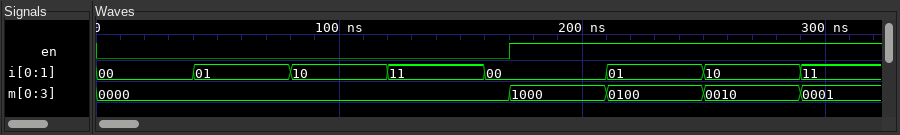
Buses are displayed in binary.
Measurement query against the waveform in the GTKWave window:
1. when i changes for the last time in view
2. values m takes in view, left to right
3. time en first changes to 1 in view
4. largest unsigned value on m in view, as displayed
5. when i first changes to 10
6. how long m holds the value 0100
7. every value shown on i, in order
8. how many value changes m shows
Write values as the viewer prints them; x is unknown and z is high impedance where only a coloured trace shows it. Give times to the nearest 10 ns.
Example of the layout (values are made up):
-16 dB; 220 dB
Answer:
290 ns; 0000, 1000, 0100, 0010, 0001; 170 ns; 1000; 80 ns; 40 ns; 00, 01, 10, 11, 00, 01, 10, 11; 4
